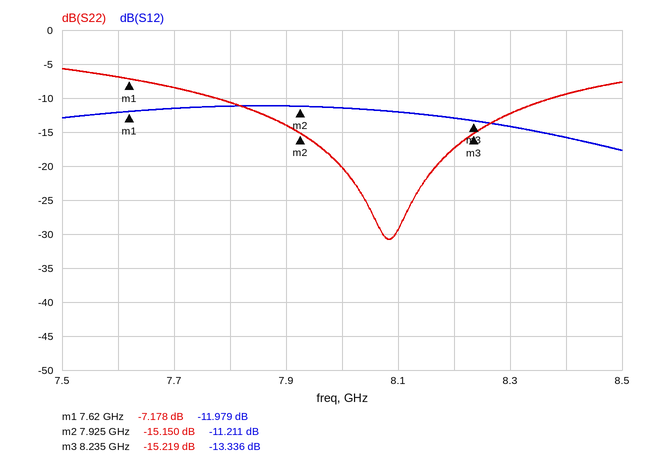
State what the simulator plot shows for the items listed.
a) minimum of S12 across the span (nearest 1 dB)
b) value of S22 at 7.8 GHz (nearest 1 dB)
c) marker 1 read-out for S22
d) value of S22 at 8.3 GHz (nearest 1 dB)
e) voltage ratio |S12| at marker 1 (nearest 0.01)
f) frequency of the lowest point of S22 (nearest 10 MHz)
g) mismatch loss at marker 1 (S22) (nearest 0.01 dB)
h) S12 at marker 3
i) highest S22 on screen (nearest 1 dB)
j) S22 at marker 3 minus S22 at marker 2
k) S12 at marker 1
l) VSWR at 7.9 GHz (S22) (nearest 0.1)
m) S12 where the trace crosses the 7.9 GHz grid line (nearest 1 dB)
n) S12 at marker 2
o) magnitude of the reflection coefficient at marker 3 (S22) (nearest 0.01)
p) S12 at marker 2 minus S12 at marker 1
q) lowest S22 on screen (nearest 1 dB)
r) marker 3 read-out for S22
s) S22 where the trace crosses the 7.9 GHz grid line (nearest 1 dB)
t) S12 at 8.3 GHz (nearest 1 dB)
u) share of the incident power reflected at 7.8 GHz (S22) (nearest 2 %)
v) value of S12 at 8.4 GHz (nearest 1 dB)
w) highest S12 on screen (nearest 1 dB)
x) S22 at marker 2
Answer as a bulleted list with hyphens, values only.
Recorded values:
- -18 dB
- -11 dB
- -7.178 dB
- -12 dB
- 0.25
- 8.08 GHz
- 0.92 dB
- -13.336 dB
- -6 dB
- -0.069 dB
- -11.979 dB
- 1.5
- -11 dB
- -11.211 dB
- 0.17
- 0.768 dB
- -31 dB
- -15.219 dB
- -14 dB
- -14 dB
- 8 %
- -16 dB
- -11 dB
- -15.150 dB
